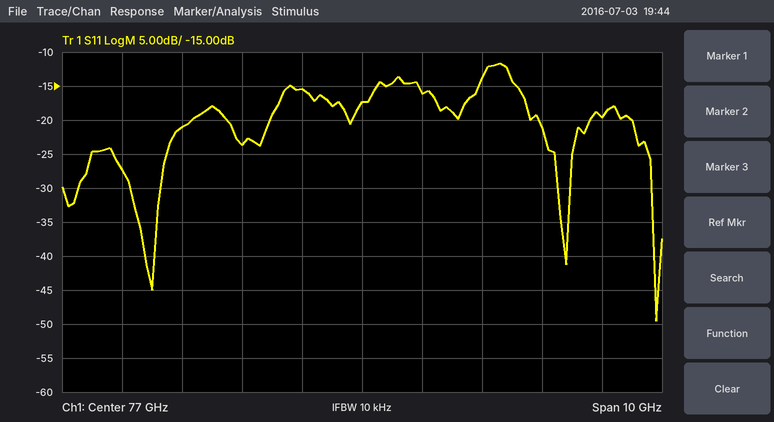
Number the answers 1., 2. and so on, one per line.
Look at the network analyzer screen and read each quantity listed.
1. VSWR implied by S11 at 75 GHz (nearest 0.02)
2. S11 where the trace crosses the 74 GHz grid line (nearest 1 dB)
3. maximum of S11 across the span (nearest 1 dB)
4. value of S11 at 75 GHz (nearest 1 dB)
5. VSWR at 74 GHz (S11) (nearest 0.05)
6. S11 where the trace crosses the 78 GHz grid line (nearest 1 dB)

1. 1.14
2. -21 dB
3. -12 dB
4. -24 dB
5. 1.20
6. -16 dB
